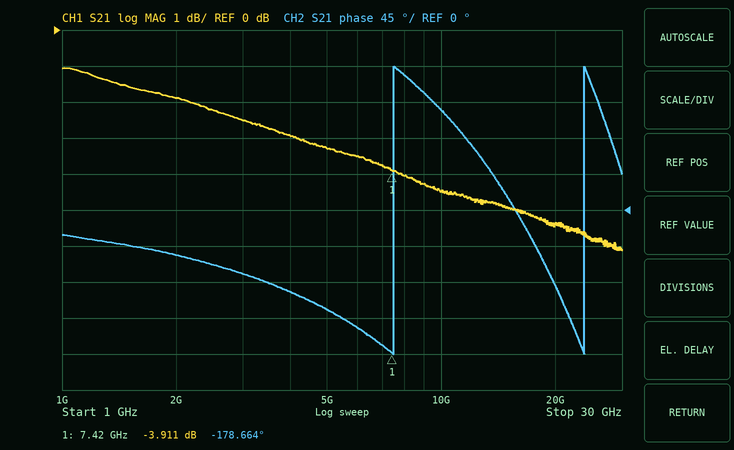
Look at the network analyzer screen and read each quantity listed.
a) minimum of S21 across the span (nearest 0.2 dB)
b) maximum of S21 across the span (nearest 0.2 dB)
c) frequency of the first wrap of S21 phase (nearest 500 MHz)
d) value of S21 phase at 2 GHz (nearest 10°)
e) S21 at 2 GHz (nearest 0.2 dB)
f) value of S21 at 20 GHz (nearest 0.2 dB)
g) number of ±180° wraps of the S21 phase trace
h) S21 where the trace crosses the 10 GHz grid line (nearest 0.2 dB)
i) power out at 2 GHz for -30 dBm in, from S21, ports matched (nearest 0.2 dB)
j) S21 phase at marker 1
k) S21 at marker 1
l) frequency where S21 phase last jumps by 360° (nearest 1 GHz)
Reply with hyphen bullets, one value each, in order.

- -6.2 dB
- -1.0 dB
- 7.5 GHz
- -60°
- -1.8 dB
- -5.4 dB
- 2
- -4.4 dB
- -31.8 dBm
- -178.664°
- -3.911 dB
- 24 GHz
